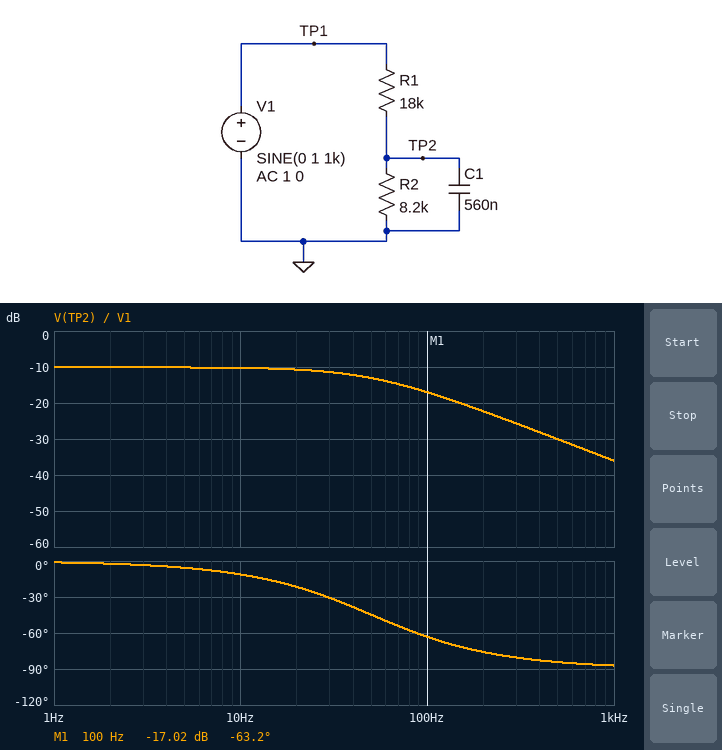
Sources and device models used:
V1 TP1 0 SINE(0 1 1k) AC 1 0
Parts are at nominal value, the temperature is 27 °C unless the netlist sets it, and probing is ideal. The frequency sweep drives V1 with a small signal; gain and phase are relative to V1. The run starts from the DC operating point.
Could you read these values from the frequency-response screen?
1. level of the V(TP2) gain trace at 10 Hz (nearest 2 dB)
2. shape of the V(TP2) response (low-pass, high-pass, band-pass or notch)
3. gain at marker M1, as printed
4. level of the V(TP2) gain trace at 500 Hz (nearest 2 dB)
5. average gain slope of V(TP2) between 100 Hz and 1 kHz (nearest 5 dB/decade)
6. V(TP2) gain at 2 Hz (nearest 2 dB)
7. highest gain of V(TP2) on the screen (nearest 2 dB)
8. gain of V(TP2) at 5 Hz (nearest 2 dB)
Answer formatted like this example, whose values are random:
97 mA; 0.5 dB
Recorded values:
-10 dB; low-pass; -17.02 dB; -30 dB; -20 dB/decade; -10 dB; -10 dB; -10 dB
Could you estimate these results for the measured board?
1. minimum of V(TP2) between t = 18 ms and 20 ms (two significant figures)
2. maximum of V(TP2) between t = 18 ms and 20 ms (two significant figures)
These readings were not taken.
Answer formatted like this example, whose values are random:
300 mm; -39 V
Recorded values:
-16 mV; 16 mV
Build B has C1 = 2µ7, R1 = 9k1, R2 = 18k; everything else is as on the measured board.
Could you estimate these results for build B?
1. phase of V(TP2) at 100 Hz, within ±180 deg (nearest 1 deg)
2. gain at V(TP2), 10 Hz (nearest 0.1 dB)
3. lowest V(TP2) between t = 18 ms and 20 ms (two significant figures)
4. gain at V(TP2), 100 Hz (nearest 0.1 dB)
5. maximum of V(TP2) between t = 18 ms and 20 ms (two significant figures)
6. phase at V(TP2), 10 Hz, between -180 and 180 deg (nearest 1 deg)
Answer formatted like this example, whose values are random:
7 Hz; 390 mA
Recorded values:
-84 deg; -6.7 dB; -4.6 mV; -23.8 dB; 8.6 mV; -46 deg
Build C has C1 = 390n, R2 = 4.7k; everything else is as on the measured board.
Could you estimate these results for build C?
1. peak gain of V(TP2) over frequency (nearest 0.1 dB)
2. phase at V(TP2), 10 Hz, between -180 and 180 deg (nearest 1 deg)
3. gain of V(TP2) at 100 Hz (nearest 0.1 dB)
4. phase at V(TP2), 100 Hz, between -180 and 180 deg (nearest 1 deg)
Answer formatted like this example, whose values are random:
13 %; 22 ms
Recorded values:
-13.7 dB; -5 deg; -16.3 dB; -42 deg
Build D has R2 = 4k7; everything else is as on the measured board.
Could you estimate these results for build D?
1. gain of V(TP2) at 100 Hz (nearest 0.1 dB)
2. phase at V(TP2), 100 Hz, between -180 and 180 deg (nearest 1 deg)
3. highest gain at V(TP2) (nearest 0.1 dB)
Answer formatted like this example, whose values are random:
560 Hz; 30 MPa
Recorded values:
-18.0 dB; -53 deg; -13.7 dB
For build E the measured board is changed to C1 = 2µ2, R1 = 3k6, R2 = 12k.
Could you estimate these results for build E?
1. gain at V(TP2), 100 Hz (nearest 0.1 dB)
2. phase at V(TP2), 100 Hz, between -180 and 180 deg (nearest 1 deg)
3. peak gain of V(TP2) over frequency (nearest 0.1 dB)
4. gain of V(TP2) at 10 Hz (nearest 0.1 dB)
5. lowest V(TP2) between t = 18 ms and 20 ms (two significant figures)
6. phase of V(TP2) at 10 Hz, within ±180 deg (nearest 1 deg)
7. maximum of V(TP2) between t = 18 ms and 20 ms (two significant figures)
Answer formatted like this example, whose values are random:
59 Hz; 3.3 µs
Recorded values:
-14.2 dB; -75 deg; -2.3 dB; -2.9 dB; -19 mV; -21 deg; 21 mV
